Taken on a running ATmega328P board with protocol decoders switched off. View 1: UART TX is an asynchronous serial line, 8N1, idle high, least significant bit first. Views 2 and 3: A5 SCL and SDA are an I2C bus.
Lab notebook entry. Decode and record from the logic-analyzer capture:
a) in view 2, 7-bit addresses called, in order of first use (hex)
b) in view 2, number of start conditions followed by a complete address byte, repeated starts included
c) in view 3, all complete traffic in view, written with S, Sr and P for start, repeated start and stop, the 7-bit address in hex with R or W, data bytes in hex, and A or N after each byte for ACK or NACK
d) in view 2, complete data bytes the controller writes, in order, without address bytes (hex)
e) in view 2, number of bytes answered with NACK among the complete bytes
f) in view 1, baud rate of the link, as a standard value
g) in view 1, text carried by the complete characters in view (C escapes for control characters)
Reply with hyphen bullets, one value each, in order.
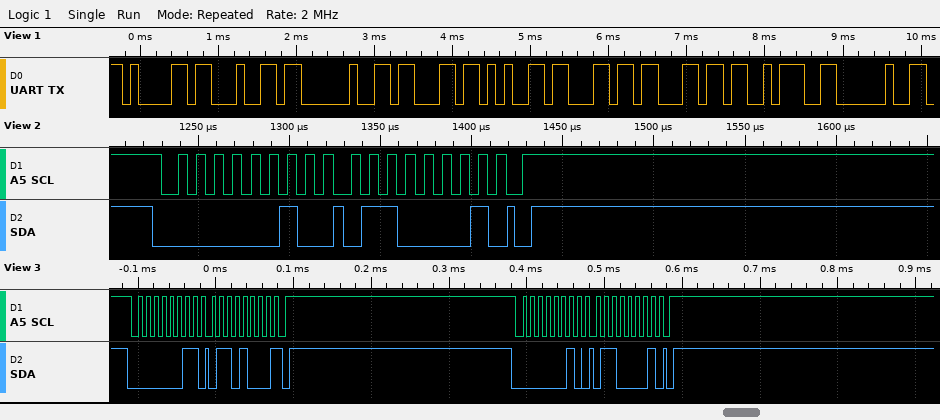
- 0x01
- 1
- S 01R A 68 N P S 01W A 61 A P
- 61
- 0
- 9600 baud
- "ad cell: "
